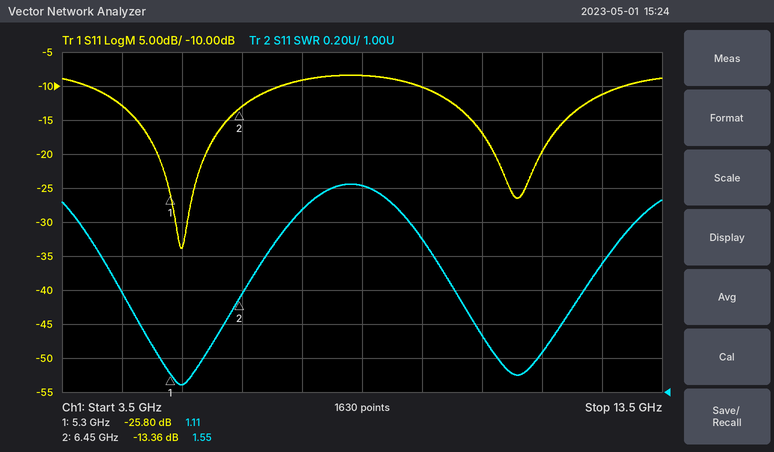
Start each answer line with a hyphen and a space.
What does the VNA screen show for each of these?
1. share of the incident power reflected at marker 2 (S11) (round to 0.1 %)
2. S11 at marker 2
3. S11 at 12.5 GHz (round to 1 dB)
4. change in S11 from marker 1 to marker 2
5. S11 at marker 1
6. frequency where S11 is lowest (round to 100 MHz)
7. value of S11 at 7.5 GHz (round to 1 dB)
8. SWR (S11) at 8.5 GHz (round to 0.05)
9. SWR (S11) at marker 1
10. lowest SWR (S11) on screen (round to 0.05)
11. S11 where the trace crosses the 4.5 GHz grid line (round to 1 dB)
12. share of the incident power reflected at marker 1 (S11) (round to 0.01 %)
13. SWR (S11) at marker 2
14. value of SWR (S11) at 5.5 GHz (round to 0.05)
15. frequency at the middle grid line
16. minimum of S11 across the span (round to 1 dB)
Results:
- 4.6 %
- -13.36 dB
- -11 dB
- 12.44 dB
- -25.80 dB
- 5.5 GHz
- -9 dB
- 2.20
- 1.11
- 1.05
- -13 dB
- 0.26 %
- 1.55
- 1.05
- 8.5 GHz
- -34 dB
